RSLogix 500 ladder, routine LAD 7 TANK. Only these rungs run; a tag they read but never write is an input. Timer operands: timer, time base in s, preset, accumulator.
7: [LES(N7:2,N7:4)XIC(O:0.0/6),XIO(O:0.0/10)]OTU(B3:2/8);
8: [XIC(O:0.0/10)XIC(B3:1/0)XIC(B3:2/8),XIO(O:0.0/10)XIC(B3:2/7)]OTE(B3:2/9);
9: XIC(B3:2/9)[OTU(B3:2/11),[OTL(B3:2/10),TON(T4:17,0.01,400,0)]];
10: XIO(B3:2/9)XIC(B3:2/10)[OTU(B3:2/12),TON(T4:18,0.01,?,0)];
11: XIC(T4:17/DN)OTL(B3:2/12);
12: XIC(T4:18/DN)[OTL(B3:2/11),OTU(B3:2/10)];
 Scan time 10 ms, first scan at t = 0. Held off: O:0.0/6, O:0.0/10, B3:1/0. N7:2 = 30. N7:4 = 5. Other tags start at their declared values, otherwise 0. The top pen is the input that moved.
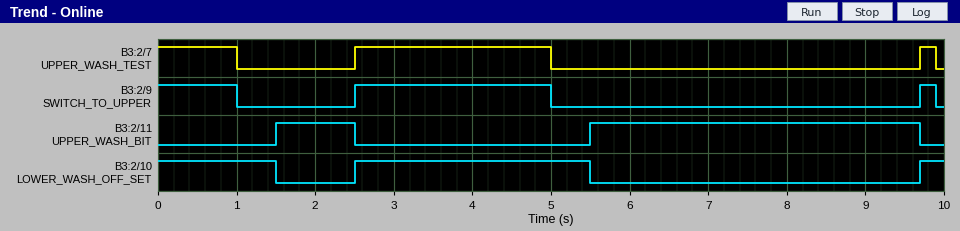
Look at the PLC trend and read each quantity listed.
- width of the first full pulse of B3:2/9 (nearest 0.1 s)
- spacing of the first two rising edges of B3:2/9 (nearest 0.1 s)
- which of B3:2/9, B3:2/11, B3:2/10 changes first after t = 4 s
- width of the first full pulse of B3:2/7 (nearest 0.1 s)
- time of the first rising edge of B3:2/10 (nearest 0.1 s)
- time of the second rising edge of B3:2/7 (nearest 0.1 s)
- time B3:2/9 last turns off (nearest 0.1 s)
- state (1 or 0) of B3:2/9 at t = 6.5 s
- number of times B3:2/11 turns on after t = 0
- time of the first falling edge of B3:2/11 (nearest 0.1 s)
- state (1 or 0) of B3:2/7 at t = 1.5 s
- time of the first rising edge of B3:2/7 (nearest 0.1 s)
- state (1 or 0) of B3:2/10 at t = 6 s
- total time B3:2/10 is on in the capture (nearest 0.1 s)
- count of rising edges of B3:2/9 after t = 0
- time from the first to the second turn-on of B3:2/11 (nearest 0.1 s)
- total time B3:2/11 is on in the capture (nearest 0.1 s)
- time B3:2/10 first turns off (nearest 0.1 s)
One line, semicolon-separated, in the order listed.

2.5 s; 7.2 s; B3:2/9; 2.5 s; 2.5 s; 9.7 s; 9.9 s; 0; 2; 2.5 s; 0; 2.5 s; 0; 4.8 s; 2; 4.0 s; 5.2 s; 1.5 s
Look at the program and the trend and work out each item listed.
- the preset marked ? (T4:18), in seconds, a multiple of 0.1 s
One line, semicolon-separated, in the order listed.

0.5 s
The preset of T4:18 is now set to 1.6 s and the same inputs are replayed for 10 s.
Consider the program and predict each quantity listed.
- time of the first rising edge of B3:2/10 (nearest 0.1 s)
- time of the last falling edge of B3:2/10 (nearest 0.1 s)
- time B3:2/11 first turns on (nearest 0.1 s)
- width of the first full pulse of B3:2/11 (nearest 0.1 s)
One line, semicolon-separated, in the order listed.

9.7 s; 6.6 s; 6.6 s; 3.1 s
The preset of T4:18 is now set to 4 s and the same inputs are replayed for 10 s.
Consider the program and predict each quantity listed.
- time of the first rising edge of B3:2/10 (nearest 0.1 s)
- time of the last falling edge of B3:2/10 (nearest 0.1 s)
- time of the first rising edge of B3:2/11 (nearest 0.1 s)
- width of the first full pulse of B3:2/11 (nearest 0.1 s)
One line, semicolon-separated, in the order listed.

9.7 s; 9.0 s; 9.0 s; 0.7 s
